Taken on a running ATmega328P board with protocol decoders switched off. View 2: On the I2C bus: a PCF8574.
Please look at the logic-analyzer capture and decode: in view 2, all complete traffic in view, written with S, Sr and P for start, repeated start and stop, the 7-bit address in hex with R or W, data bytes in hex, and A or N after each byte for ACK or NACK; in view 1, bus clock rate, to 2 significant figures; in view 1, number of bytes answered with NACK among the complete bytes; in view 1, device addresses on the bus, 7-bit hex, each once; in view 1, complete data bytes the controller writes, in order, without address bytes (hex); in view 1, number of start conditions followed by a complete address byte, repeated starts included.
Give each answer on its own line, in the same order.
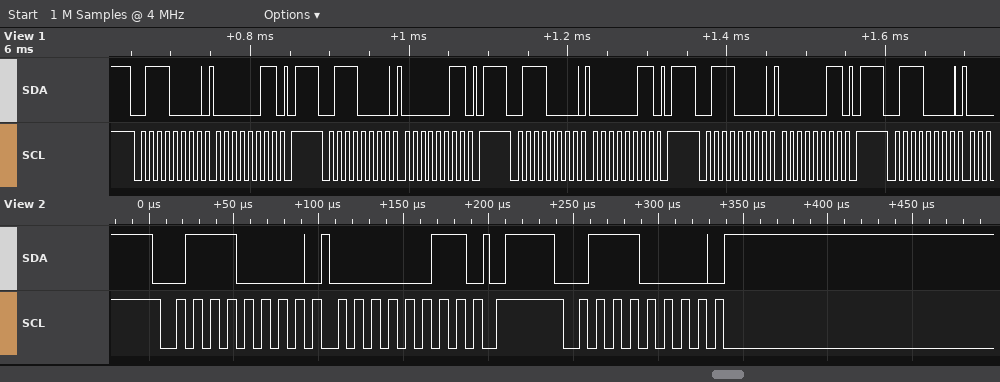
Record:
S 38W A 03 A P S 38W A
100 kHz
0
0x38
03 03 03 03
5
